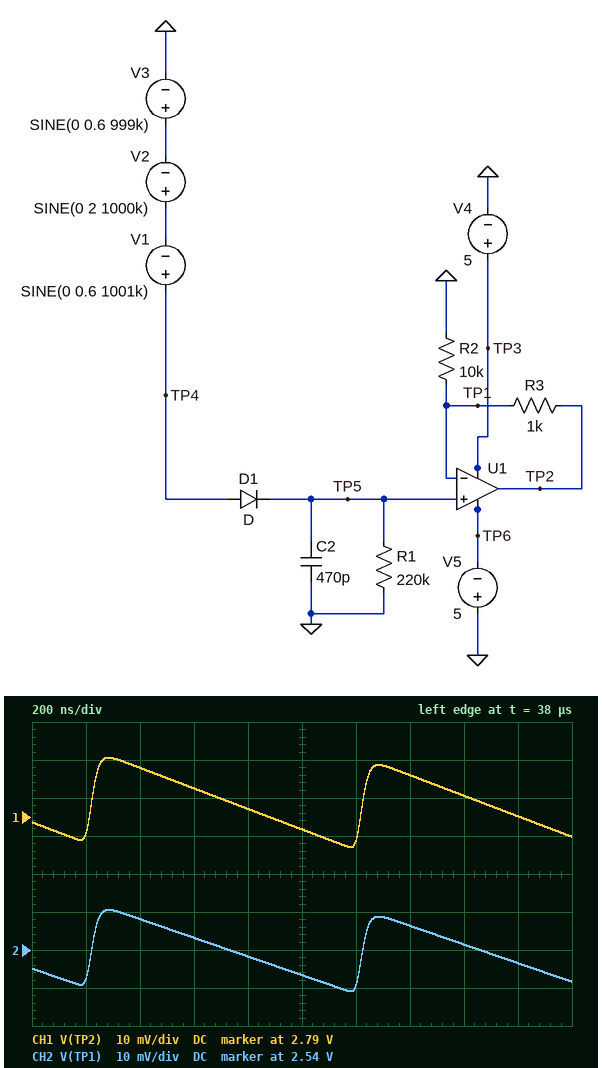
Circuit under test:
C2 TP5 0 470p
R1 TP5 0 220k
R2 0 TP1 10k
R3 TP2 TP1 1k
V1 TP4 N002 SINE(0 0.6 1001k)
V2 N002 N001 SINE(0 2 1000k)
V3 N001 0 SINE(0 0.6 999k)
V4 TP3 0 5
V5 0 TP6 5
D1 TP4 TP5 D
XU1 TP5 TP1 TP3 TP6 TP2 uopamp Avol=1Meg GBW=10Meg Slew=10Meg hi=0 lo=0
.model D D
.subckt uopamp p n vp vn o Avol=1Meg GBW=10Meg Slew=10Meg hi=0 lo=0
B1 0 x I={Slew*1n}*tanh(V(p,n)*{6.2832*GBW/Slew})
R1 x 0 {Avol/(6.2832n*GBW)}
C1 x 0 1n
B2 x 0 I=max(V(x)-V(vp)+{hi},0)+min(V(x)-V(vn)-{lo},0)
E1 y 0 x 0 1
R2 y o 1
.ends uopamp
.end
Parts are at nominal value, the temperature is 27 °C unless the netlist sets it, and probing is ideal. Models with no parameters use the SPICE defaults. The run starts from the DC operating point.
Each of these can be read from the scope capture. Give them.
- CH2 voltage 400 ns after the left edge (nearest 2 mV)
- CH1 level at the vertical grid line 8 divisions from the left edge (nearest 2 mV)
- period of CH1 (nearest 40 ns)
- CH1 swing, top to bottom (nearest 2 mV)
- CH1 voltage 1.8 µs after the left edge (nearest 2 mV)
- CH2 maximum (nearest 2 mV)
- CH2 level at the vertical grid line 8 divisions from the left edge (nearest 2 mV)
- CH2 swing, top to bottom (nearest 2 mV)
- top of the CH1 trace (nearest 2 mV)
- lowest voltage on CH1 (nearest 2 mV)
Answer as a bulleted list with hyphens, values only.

- 2.548 V
- 2.796 V
- 1.00 µs
- 24 mV
- 2.790 V
- 2.550 V
- 2.542 V
- 22 mV
- 2.806 V
- 2.782 V
